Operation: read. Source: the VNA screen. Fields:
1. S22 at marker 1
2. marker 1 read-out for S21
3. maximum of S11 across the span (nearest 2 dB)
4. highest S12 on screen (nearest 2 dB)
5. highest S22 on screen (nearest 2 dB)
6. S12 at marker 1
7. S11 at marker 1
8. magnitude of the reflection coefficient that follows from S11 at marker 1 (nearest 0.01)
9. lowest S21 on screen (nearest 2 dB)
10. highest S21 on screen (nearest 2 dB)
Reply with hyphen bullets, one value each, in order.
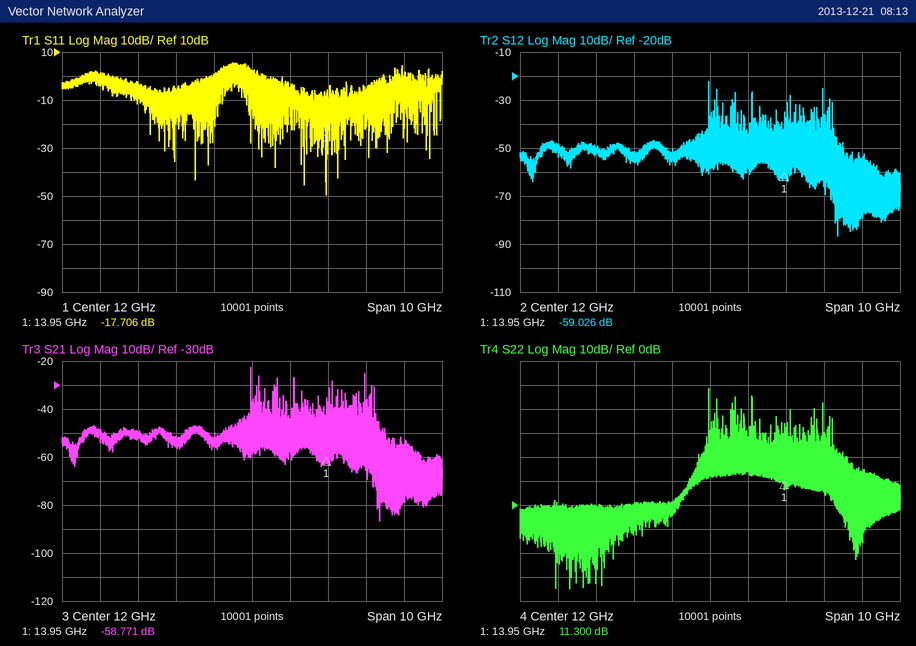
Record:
- 11.300 dB
- -58.771 dB
- 6 dB
- -22 dB
- 48 dB
- -59.026 dB
- -17.706 dB
- 0.13
- -86 dB
- -22 dB
